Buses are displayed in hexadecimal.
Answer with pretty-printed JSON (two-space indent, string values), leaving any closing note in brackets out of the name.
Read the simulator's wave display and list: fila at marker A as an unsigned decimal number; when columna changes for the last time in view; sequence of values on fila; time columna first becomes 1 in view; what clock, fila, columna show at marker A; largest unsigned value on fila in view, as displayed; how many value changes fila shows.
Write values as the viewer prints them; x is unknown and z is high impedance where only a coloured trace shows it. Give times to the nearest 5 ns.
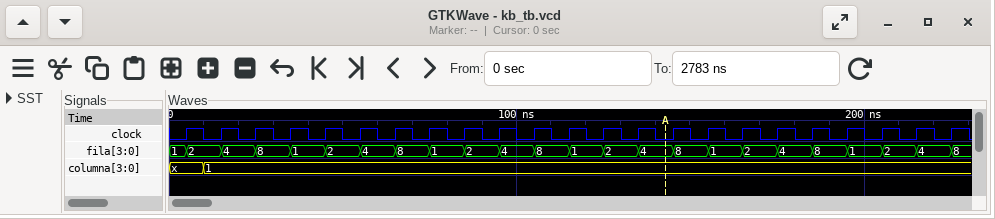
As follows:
{
  "fila at marker A as an unsigned decimal number": "4",
  "when columna changes for the last time in view": "10 ns",
  "sequence of values on fila": "1, 2, 4, 8, 1, 2, 4, 8, 1, 2, 4, 8, 1, 2, 4, 8, 1, 2, 4, 8, 1, 2, 4, 8",
  "time columna first becomes 1 in view": "10 ns",
  "what clock, fila, columna show at marker A": "clock=0, fila=4, columna=1",
  "largest unsigned value on fila in view, as displayed": "8",
  "how many value changes fila shows": "23"
}
